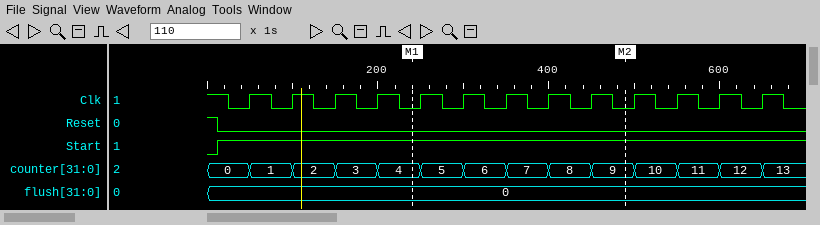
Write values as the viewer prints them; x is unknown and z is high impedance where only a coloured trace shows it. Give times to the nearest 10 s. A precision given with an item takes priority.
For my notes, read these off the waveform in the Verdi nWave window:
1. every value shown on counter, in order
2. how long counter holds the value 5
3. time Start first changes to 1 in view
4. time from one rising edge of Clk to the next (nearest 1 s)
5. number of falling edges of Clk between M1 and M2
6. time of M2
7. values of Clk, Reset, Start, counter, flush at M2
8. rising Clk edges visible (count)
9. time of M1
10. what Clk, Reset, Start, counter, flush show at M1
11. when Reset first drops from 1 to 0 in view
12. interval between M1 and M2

0, 1, 2, 3, 4, 5, 6, 7, 8, 9, 10, 11, 12, 13
50 s
10 s
50 s
5
490 s
Clk=0, Reset=0, Start=1, counter=9, flush=0
13
240 s
Clk=0, Reset=0, Start=1, counter=4, flush=0
10 s
250 s
